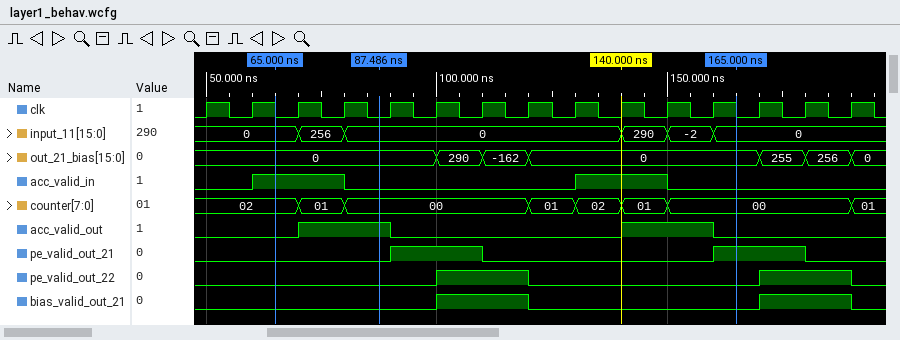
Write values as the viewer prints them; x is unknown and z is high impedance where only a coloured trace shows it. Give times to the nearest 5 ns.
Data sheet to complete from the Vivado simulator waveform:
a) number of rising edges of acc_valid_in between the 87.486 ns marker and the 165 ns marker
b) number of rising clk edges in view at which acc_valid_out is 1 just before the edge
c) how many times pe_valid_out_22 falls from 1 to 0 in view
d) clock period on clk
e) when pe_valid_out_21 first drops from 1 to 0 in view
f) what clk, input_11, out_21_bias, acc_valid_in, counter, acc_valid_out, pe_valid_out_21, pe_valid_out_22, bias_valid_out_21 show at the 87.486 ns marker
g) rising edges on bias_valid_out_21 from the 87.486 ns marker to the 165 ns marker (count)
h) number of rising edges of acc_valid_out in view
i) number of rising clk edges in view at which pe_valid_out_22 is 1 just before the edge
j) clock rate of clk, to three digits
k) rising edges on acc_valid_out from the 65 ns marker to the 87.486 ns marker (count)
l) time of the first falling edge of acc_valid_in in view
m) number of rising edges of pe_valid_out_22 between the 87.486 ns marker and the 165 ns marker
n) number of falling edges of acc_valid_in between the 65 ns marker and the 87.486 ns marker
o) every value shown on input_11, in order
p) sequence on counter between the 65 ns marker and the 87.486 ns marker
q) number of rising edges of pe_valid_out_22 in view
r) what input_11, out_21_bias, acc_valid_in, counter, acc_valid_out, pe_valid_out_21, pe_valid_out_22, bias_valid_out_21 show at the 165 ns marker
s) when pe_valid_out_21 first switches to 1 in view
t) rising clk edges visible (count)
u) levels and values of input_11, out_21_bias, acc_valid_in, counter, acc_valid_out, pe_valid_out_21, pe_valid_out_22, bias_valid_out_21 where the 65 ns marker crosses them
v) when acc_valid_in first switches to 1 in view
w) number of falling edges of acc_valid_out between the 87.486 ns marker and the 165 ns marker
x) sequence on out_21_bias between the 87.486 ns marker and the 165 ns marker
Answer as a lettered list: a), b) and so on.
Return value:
a) 1
b) 4
c) 2
d) 10 ns
e) 110 ns
f) clk=0, input_11=0, out_21_bias=0, acc_valid_in=0, counter=00, acc_valid_out=1, pe_valid_out_21=0, pe_valid_out_22=0, bias_valid_out_21=0
g) 1
h) 2
i) 4
j) 100 MHz
k) 1
l) 80 ns
m) 1
n) 1
o) 0, 256, 0, 290, -2, 0
p) 02, 01, 00
q) 2
r) input_11=0, out_21_bias=0, acc_valid_in=0, counter=00, acc_valid_out=0, pe_valid_out_21=1, pe_valid_out_22=0, bias_valid_out_21=0
s) 90 ns
t) 15
u) input_11=0, out_21_bias=0, acc_valid_in=1, counter=02, acc_valid_out=0, pe_valid_out_21=0, pe_valid_out_22=0, bias_valid_out_21=0
v) 60 ns
w) 2
x) 0, 290, -162, 0
